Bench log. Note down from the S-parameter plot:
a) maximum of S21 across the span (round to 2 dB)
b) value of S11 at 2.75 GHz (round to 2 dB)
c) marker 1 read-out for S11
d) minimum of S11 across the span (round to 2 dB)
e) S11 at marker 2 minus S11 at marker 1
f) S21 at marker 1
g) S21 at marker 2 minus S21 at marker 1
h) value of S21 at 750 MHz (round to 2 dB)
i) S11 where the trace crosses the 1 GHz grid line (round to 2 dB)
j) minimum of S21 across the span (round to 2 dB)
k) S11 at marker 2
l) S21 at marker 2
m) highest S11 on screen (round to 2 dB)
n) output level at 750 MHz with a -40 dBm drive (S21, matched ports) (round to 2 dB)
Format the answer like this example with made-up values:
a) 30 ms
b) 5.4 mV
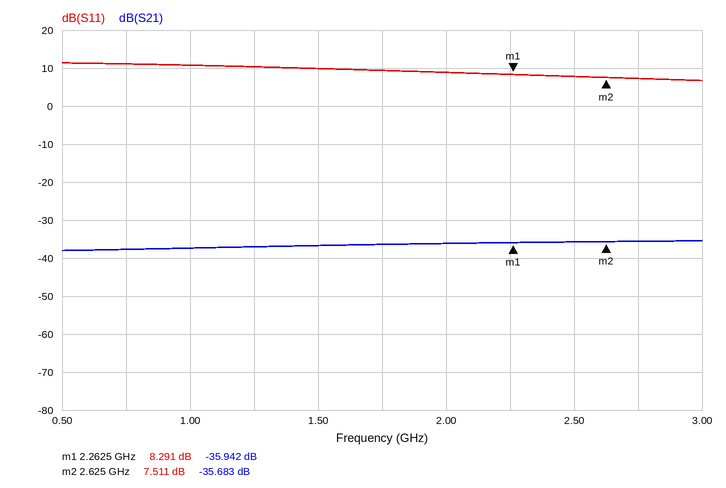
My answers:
a) -36 dB
b) 8 dB
c) 8.291 dB
d) 6 dB
e) -0.780 dB
f) -35.942 dB
g) 0.259 dB
h) -38 dB
i) 10 dB
j) -38 dB
k) 7.511 dB
l) -35.683 dB
m) 12 dB
n) -78 dBm
